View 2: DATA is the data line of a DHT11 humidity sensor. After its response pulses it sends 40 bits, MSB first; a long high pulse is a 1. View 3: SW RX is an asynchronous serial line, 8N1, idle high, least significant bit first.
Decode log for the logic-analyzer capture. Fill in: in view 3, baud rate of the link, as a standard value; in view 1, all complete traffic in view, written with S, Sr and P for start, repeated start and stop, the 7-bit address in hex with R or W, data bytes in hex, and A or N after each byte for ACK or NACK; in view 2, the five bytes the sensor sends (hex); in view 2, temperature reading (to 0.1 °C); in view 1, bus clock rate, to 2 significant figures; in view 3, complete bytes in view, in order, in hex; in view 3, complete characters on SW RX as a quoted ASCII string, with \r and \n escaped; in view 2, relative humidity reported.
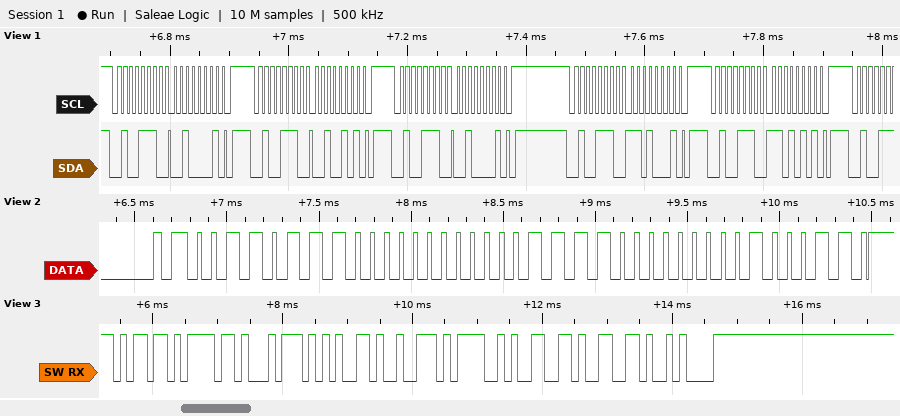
9600 baud
S 27W A 21 A P S 27W A 25 A P S 27W A 21 A P S 27W A D1 A P S 27W A D5 A P
37 00 0F 00 46
15.0 °C
100 kHz
6D 6F 74 65 72 4F 66 66 0A
"moterOff\n"
55 %
